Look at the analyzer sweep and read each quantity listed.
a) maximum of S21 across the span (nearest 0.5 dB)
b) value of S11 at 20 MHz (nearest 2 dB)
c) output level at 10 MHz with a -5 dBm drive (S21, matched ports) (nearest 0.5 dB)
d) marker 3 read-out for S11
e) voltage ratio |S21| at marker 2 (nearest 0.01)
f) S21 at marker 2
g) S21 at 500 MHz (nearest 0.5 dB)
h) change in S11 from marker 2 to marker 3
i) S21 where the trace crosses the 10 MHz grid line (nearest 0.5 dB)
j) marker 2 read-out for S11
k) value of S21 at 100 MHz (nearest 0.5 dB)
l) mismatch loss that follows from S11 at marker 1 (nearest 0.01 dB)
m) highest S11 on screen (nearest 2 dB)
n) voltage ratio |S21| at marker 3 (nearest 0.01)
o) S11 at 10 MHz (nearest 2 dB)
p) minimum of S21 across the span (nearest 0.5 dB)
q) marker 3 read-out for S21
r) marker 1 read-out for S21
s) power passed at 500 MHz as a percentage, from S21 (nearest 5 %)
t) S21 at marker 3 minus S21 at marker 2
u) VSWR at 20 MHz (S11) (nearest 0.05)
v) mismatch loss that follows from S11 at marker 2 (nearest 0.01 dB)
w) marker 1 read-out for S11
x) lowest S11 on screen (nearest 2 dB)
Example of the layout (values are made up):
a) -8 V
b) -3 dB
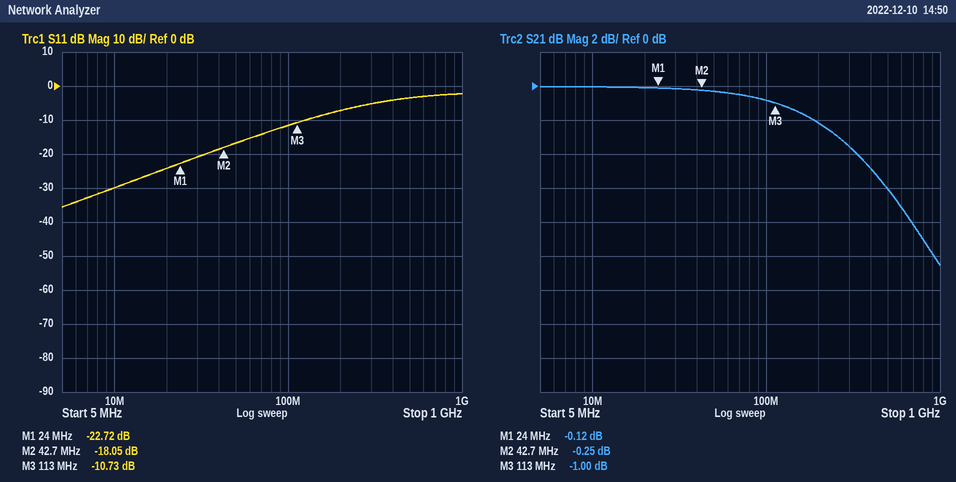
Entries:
a) 0.0 dB
b) -24 dB
c) -5.0 dBm
d) -10.73 dB
e) 0.97
f) -0.25 dB
g) -6.0 dB
h) 7.32 dB
i) 0.0 dB
j) -18.05 dB
k) -1.0 dB
l) 0.02 dB
m) -2 dB
n) 0.89
o) -30 dB
p) -10.5 dB
q) -1.00 dB
r) -0.12 dB
s) 25 %
t) -0.75 dB
u) 1.15
v) 0.07 dB
w) -22.72 dB
x) -36 dB
